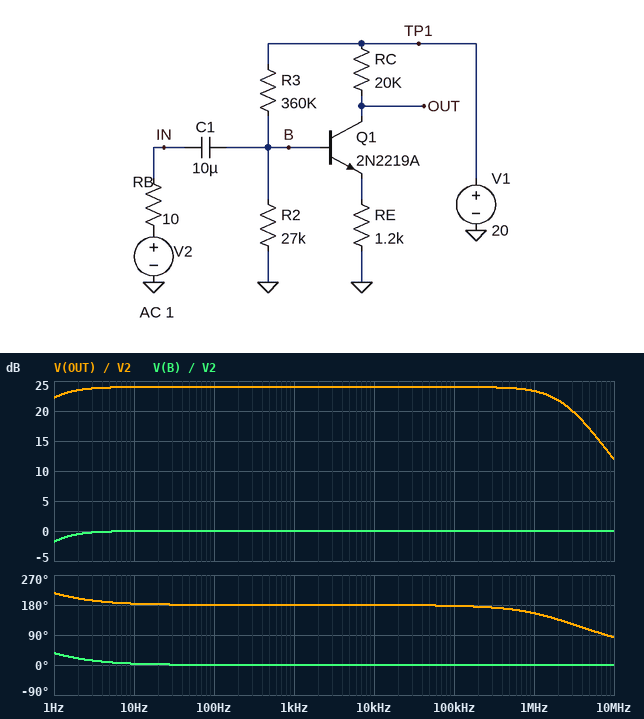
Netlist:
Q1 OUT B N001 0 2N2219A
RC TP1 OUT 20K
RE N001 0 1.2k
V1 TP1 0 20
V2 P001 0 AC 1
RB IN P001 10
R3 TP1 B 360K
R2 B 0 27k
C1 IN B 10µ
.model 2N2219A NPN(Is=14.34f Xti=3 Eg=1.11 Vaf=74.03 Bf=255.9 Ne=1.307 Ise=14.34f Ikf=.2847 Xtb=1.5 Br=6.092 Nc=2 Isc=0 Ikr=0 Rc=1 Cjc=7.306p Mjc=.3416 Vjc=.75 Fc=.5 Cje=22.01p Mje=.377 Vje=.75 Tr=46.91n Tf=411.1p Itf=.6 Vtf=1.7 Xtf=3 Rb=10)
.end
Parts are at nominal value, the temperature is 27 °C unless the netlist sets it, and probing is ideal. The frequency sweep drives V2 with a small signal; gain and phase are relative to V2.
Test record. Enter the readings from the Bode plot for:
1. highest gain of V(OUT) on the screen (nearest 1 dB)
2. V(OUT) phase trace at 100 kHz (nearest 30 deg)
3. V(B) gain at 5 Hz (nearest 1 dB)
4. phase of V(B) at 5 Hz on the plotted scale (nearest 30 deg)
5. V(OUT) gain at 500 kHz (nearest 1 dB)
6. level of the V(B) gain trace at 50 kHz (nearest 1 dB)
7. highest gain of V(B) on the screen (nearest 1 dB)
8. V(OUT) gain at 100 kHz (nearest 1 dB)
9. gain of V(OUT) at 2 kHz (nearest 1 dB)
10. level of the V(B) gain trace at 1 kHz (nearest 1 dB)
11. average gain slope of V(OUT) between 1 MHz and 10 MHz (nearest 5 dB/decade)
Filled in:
24 dB
180 deg
0 dB
0 deg
24 dB
0 dB
0 dB
24 dB
24 dB
0 dB
-10 dB/decade
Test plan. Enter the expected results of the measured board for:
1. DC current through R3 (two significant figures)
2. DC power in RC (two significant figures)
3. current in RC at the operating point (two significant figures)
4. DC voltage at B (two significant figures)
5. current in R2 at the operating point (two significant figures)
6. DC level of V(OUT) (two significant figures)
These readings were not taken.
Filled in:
52 µA
6.2 mW
560 µA
1.3 V
48 µA
8.8 V
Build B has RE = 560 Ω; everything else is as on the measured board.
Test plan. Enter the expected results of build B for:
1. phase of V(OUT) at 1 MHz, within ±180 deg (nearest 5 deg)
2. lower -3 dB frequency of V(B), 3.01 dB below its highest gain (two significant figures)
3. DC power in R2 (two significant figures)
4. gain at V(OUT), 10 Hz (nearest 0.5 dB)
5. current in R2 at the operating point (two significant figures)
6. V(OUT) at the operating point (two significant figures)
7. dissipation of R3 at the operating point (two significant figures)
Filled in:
120 deg
14 Hz
53 µW
17.5 dB
44 µA
670 mV
980 µW
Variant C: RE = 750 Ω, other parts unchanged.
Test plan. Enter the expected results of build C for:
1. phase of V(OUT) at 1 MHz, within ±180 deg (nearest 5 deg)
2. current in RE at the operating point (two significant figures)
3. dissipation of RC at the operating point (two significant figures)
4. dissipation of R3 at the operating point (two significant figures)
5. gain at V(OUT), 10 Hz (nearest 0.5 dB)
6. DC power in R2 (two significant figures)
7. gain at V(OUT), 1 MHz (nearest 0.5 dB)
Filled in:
150 deg
820 µA
13 mW
980 µW
28.0 dB
59 µW
27.0 dB
